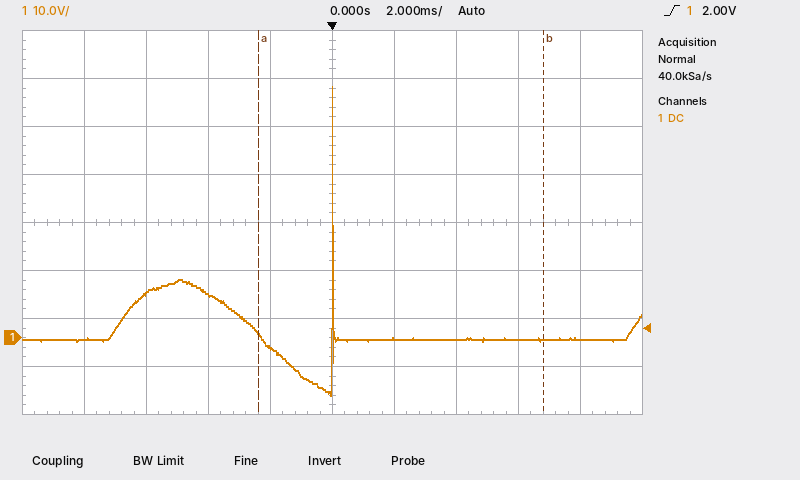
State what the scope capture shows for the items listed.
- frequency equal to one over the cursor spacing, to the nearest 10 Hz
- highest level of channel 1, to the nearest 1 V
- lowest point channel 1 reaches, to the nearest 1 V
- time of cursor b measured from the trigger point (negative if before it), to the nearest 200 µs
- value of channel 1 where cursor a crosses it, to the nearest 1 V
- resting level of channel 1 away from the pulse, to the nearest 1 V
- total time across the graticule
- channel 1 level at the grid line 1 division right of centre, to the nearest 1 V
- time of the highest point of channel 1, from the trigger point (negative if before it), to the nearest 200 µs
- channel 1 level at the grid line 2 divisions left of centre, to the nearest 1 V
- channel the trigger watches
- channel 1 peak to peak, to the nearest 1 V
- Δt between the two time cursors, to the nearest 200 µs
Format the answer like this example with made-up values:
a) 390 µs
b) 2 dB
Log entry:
a) 110 Hz
b) 52 V
c) -12 V
d) +6.8 ms
e) 1 V
f) 0 V
g) 20 ms
h) 0 V
i) 0.0 ms
j) 9 V
k) channel 1
l) 64 V
m) 9.2 ms
